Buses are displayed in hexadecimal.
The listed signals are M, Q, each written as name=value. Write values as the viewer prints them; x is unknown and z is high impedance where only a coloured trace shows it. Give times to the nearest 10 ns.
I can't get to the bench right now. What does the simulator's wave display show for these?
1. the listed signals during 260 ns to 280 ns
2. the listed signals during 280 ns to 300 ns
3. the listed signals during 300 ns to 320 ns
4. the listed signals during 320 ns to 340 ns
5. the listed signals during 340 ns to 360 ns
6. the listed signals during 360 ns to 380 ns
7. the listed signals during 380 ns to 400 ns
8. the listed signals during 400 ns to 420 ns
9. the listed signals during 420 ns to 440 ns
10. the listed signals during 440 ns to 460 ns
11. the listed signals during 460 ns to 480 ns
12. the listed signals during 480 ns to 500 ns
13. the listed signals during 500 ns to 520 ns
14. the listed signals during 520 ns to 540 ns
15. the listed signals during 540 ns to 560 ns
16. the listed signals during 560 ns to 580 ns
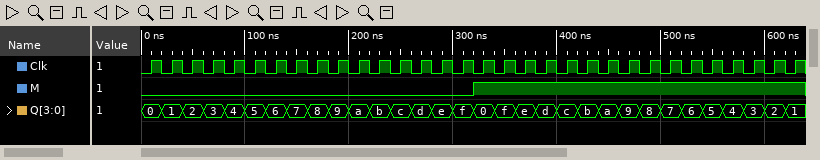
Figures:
M=0, Q=d
M=0, Q=e
M=0, Q=f
M=1, Q=0
M=1, Q=f
M=1, Q=e
M=1, Q=d
M=1, Q=c
M=1, Q=b
M=1, Q=a
M=1, Q=9
M=1, Q=8
M=1, Q=7
M=1, Q=6
M=1, Q=5
M=1, Q=4
